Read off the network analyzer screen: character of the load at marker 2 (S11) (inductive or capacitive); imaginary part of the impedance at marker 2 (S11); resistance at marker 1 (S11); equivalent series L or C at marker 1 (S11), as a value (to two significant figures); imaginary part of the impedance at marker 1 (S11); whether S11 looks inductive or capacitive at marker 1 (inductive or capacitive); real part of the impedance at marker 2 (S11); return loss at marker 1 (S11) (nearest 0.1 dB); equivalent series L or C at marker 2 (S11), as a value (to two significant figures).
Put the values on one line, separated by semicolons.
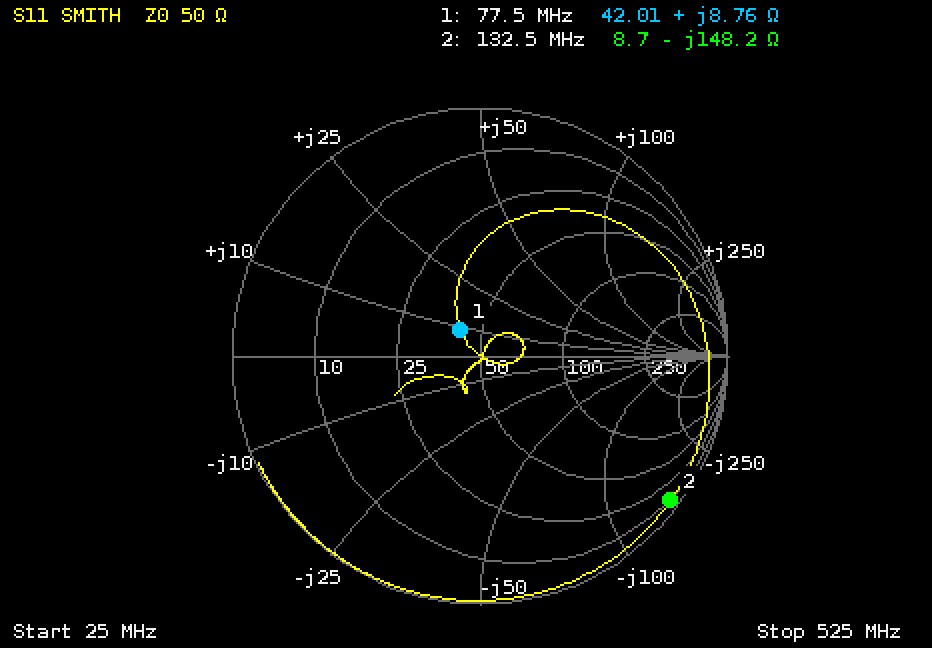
capacitive; -148.2 Ω; 42.01 Ω; 18 nH; +8.76 Ω; inductive; 8.7 Ω; 17.8 dB; 8.1 pF
